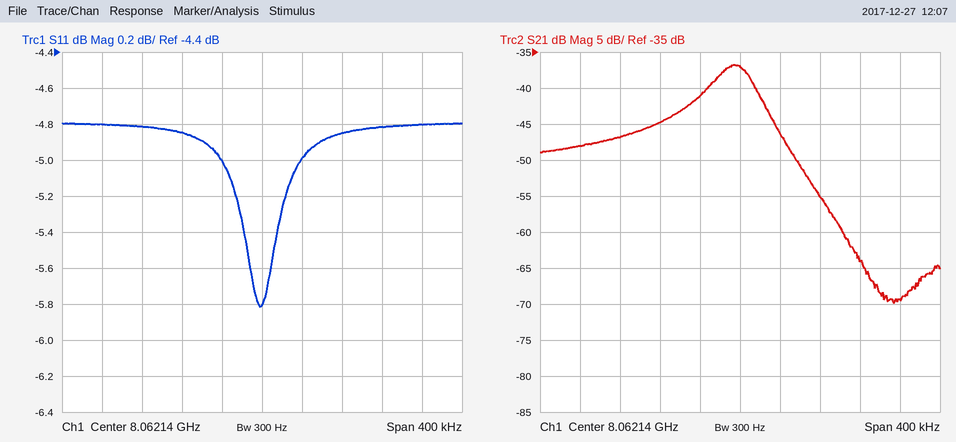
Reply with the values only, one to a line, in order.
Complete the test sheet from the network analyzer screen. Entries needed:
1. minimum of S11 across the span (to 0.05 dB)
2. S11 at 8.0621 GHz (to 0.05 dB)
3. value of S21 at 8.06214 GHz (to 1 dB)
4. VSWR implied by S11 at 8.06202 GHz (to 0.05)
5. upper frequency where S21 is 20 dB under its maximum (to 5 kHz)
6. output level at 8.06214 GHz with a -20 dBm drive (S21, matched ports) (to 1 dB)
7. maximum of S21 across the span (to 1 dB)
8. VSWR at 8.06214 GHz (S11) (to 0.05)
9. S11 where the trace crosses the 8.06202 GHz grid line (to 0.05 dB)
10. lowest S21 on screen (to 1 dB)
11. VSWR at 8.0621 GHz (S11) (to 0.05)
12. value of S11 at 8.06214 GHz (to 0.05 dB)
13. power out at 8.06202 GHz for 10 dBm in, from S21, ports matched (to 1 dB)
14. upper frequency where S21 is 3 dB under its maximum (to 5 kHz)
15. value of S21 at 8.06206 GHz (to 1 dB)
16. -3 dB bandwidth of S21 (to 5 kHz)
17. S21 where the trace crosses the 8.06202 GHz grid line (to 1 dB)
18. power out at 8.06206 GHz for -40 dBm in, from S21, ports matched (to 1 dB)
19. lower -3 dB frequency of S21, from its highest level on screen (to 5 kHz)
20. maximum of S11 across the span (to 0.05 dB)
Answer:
-5.80 dB
-5.00 dB
-37 dB
3.70
8.062230 GHz
-57 dBm
-37 dB
3.10
-4.80 dB
-70 dB
3.55
-5.80 dB
-37 dBm
8.062155 GHz
-45 dB
45 kHz
-47 dB
-85 dBm
8.062110 GHz
-4.80 dB
